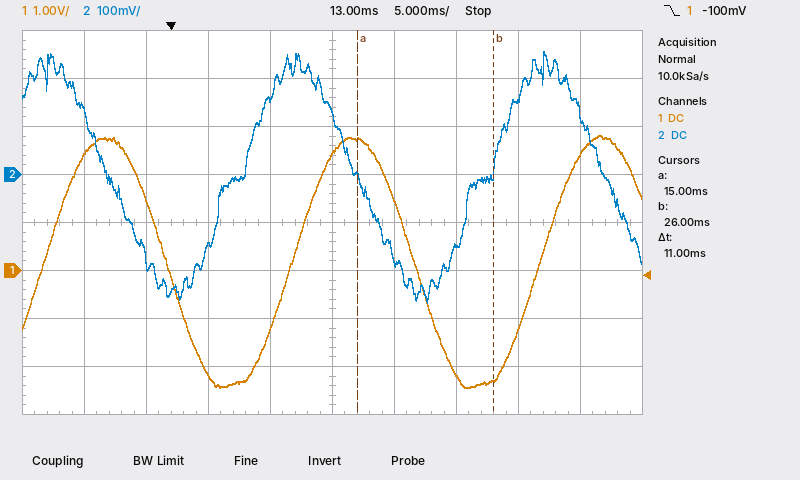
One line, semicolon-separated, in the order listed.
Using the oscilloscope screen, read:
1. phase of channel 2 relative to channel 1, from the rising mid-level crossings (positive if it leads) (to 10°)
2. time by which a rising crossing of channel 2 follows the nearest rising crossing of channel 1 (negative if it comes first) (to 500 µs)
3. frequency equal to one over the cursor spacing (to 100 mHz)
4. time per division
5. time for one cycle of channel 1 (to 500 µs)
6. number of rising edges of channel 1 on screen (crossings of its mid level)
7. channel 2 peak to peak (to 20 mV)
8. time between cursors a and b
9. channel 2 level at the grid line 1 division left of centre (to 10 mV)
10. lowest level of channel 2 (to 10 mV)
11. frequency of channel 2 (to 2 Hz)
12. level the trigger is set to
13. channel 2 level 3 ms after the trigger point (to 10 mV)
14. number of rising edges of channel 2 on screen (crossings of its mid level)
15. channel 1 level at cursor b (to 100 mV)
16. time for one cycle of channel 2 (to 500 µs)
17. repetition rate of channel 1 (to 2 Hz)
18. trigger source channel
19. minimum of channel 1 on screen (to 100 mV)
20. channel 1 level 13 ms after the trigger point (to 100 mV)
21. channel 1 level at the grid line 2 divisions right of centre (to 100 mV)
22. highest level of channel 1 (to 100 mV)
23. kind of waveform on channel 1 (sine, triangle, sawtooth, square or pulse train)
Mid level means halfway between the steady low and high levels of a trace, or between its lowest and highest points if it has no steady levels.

+70°; -4.0 ms; 90.9 Hz; 5 ms; 20.0 ms; 3; 520 mV; 11 ms; 160 mV; -270 mV; 50 Hz; -100 mV; -150 mV; 2; -2.3 V; 20.0 ms; 50 Hz; channel 1; -2.4 V; 2.4 V; -2.2 V; 2.8 V; sine
